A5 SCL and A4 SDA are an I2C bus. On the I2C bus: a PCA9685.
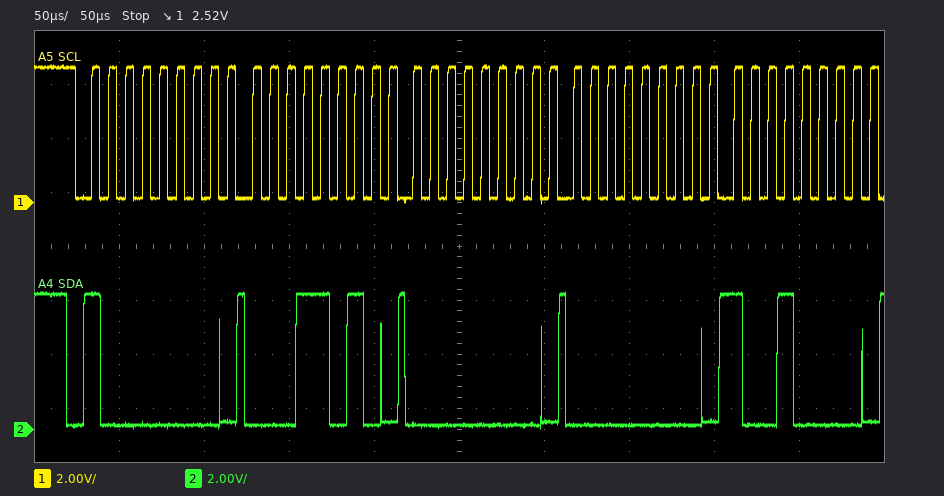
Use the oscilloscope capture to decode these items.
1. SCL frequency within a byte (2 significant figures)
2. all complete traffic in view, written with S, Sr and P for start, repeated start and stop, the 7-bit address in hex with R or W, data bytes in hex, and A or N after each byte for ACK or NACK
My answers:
100 kHz
S 40W A 1A A 00 A 00 A 90 A
